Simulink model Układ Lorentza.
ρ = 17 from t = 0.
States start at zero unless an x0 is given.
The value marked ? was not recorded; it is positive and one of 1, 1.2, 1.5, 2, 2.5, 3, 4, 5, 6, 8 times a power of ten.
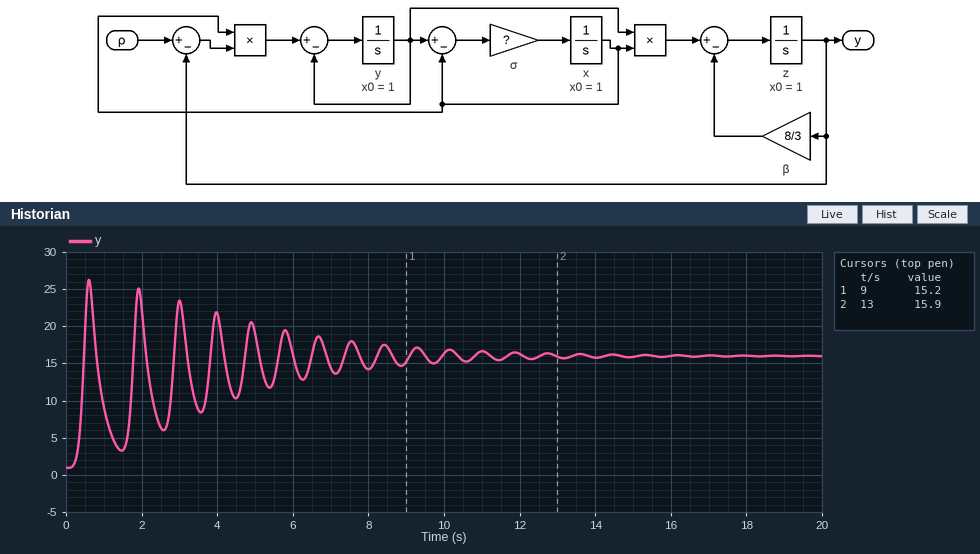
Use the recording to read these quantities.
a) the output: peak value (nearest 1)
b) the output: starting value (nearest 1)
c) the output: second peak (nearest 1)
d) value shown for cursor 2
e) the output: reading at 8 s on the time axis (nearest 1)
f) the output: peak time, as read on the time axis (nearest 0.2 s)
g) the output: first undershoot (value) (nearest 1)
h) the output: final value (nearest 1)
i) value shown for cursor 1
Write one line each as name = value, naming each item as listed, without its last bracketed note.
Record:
the output: peak value = 26
the output: starting value = 1
the output: second peak = 25
value shown for cursor 2 = 15.9
the output: reading at 8 s on the time axis = 14
the output: peak time, as read on the time axis = 0.6 s
the output: first undershoot (value) = 3
the output: final value = 16
value shown for cursor 1 = 15.2
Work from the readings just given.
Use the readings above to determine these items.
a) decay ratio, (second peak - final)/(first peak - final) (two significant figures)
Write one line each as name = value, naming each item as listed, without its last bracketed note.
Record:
decay ratio, (second peak - final)/(first peak - final) = 0.90
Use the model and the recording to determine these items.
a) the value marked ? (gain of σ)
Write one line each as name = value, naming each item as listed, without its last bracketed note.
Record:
the value marked ? = 5
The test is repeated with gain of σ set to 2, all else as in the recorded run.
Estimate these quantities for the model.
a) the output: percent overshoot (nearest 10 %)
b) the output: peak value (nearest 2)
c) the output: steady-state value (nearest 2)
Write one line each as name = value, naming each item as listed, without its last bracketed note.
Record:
the output: percent overshoot = 60 %
the output: peak value = 24
the output: steady-state value = 16
